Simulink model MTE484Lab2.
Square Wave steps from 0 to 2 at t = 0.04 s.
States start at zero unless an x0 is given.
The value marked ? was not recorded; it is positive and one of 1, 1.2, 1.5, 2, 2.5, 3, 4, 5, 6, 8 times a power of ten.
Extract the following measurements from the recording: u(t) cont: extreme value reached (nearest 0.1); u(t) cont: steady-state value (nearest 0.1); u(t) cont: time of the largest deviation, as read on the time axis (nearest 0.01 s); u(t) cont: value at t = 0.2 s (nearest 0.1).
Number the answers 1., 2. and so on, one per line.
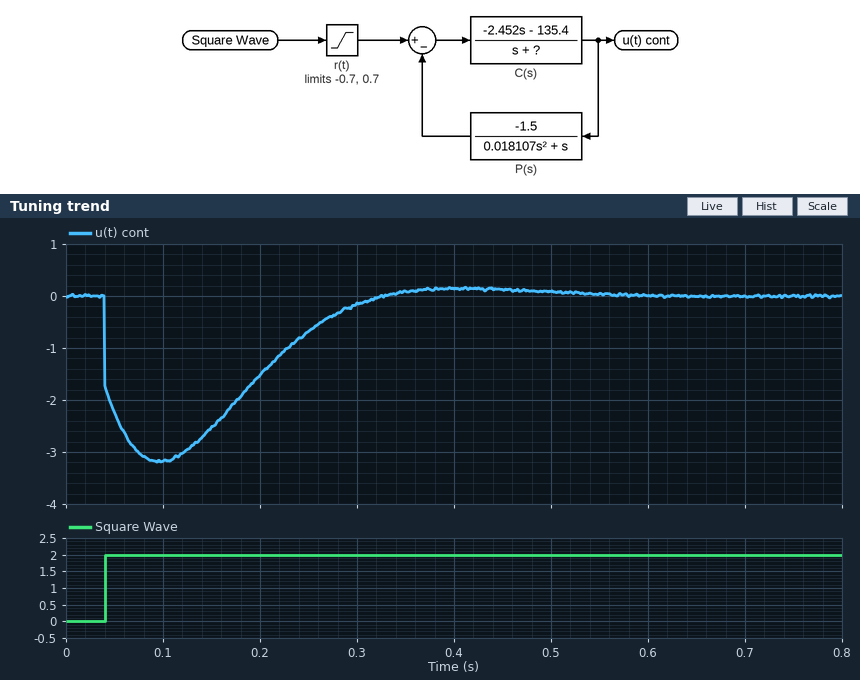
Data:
1. -3.2
2. 0.0
3. 0.10 s
4. -1.5
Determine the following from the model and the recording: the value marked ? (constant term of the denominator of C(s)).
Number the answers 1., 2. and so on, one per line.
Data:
1. 20
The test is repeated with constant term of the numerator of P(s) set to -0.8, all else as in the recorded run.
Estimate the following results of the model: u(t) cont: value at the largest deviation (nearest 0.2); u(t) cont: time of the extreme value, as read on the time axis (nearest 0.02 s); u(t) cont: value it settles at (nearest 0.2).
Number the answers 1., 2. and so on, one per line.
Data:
1. -3.6
2. 0.12 s
3. 0.0
